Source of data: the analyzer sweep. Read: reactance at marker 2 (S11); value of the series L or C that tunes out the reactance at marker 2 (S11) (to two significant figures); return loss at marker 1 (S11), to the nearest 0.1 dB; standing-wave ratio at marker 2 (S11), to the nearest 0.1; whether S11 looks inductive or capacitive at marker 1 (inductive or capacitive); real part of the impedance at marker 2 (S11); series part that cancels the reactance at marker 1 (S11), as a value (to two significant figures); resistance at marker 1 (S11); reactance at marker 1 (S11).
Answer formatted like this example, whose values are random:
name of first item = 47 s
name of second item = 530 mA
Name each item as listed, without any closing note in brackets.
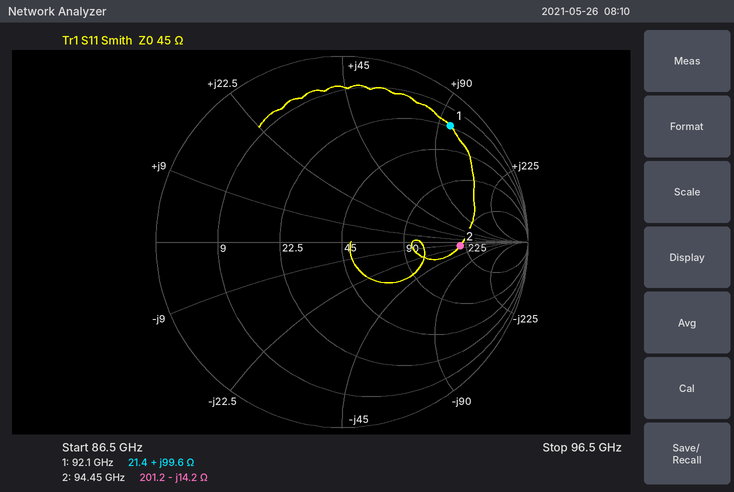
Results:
reactance at marker 2 = -14.2 Ω
value of the series L or C that tunes out the reactance at marker 2 (S11) = 24 pH
return loss at marker 1 (S11), to the nearest 0.1 dB = 1.4 dB
standing-wave ratio at marker 2 (S11), to the nearest 0.1 = 4.5
whether S11 looks inductive or capacitive at marker 1 = inductive
real part of the impedance at marker 2 = 201.2 Ω
series part that cancels the reactance at marker 1 (S11), as a value = 17 fF
resistance at marker 1 = 21.4 Ω
reactance at marker 1 = +99.6 Ω
